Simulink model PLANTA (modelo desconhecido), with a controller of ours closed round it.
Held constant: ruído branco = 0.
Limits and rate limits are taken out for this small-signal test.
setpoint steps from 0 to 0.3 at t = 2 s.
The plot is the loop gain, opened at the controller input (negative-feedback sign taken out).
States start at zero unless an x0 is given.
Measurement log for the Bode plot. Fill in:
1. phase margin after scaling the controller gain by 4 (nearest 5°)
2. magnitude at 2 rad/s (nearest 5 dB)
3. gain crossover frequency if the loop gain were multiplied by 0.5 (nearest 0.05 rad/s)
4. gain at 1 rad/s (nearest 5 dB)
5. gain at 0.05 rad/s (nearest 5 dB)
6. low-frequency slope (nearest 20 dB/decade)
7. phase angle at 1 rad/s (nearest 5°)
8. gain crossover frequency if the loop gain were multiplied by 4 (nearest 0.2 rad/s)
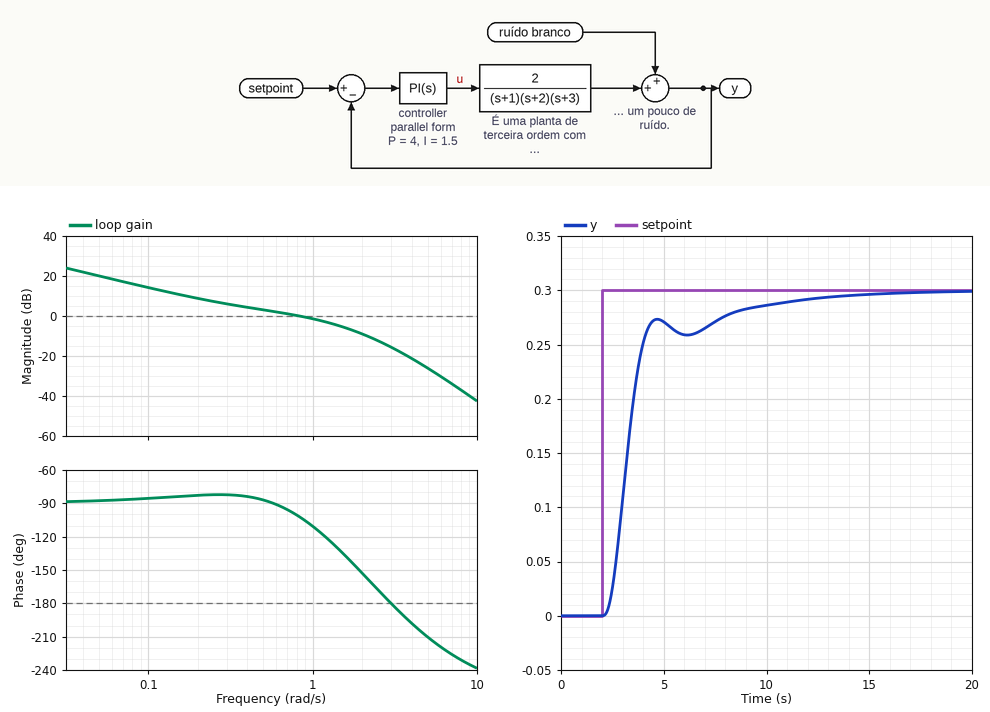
15°
-10 dB
0.30 rad/s
0 dB
20 dB
-20 dB/decade
-110°
2.4 rad/s
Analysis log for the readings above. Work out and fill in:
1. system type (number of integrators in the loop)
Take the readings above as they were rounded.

1
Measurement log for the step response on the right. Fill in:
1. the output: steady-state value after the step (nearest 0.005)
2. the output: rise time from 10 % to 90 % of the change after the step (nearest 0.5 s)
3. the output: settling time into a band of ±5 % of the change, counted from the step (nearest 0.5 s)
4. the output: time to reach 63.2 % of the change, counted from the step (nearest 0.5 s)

0.300
2.0 s
7.5 s
1.5 s
